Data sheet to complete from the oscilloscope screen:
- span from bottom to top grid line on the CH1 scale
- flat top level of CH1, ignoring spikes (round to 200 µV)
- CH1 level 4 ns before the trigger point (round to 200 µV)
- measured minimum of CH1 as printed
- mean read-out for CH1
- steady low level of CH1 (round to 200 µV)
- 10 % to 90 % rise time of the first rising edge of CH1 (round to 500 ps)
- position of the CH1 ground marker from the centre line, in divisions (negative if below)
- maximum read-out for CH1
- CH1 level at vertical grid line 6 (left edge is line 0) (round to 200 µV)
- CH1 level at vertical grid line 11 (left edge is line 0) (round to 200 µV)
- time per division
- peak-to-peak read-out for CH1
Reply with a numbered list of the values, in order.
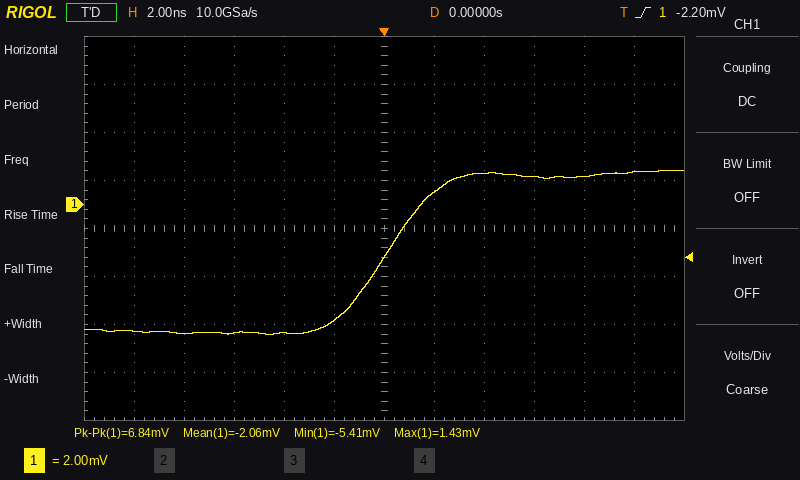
1. 16 mV
2. 1.2 mV
3. -5.4 mV
4. -5.41 mV
5. -2.06 mV
6. -5.4 mV
7. 4.0 ns
8. +0.5 div
9. 1.43 mV
10. -2.2 mV
11. 1.4 mV
12. 2 ns
13. 6.84 mV
